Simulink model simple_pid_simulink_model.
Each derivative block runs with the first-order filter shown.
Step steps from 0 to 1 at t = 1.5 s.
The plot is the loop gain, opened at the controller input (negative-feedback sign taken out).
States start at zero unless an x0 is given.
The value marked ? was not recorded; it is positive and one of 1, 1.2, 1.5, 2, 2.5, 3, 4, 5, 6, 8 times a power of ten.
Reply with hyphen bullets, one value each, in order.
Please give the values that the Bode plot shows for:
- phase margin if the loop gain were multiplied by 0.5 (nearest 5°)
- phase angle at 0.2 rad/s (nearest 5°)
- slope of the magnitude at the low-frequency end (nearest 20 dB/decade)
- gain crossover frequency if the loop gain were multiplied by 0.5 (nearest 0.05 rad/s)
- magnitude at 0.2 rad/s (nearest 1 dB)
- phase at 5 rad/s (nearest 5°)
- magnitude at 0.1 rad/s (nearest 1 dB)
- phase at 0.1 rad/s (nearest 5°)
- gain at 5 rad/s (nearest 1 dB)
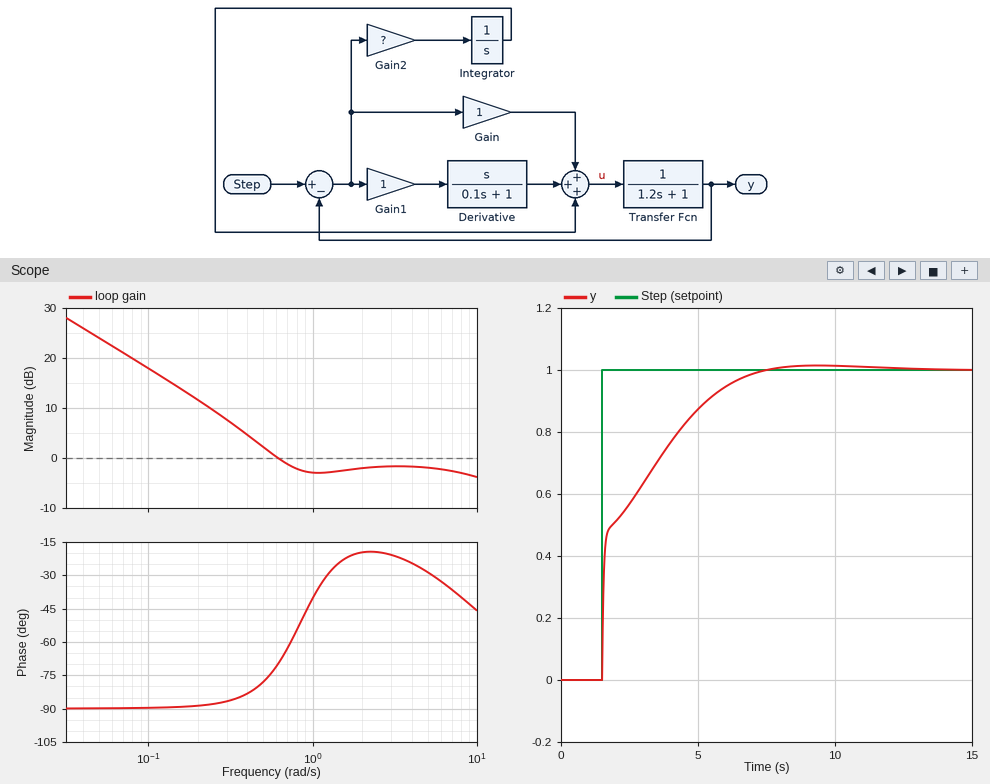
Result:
- 95°
- -90°
- -20 dB/decade
- 0.35 rad/s
- 12 dB
- -30°
- 18 dB
- -90°
- -2 dB
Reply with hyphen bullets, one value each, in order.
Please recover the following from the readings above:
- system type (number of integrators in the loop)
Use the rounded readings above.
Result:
- 1
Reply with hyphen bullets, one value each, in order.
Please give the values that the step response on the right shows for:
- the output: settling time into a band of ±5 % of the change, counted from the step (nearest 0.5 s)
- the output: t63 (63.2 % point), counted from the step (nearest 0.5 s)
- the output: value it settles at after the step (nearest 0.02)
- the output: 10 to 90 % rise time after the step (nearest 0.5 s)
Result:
- 4.5 s
- 1.5 s
- 1.00
- 4.0 s
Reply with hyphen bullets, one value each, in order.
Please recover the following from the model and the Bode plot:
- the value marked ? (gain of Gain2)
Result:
- 0.8
